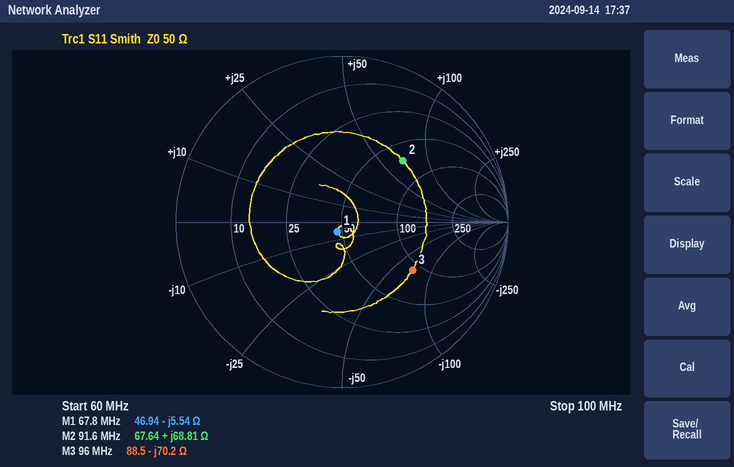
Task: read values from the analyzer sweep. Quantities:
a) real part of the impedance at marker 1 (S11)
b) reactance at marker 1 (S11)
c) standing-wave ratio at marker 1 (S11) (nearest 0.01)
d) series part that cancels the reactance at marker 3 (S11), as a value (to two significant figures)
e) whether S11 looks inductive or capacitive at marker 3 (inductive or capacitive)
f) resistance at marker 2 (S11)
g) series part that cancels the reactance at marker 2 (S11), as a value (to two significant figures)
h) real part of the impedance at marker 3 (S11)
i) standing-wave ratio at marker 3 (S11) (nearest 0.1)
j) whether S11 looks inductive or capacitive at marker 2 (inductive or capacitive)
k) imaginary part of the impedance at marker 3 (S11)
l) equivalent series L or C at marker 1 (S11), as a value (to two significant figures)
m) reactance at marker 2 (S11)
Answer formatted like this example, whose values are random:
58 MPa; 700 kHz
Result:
46.94 Ω; -5.54 Ω; 1.14; 120 nH; capacitive; 67.64 Ω; 25 pF; 88.5 Ω; 3.1; inductive; -70.2 Ω; 420 pF; +68.81 Ω
